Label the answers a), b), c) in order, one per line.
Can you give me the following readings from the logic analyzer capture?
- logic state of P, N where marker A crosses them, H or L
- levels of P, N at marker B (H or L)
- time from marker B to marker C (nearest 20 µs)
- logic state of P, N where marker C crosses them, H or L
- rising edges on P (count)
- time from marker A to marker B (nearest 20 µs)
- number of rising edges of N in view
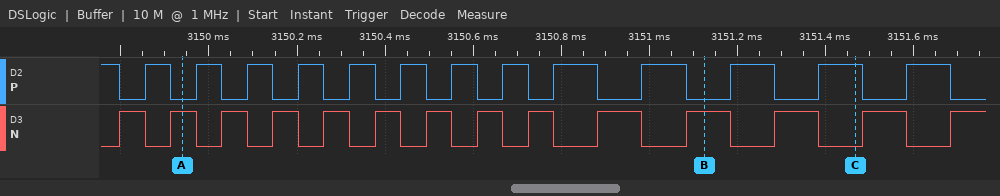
a) P=L, N=H
b) P=L, N=H
c) 340 µs
d) P=H, N=L
e) 13
f) 1180 µs
g) 14
